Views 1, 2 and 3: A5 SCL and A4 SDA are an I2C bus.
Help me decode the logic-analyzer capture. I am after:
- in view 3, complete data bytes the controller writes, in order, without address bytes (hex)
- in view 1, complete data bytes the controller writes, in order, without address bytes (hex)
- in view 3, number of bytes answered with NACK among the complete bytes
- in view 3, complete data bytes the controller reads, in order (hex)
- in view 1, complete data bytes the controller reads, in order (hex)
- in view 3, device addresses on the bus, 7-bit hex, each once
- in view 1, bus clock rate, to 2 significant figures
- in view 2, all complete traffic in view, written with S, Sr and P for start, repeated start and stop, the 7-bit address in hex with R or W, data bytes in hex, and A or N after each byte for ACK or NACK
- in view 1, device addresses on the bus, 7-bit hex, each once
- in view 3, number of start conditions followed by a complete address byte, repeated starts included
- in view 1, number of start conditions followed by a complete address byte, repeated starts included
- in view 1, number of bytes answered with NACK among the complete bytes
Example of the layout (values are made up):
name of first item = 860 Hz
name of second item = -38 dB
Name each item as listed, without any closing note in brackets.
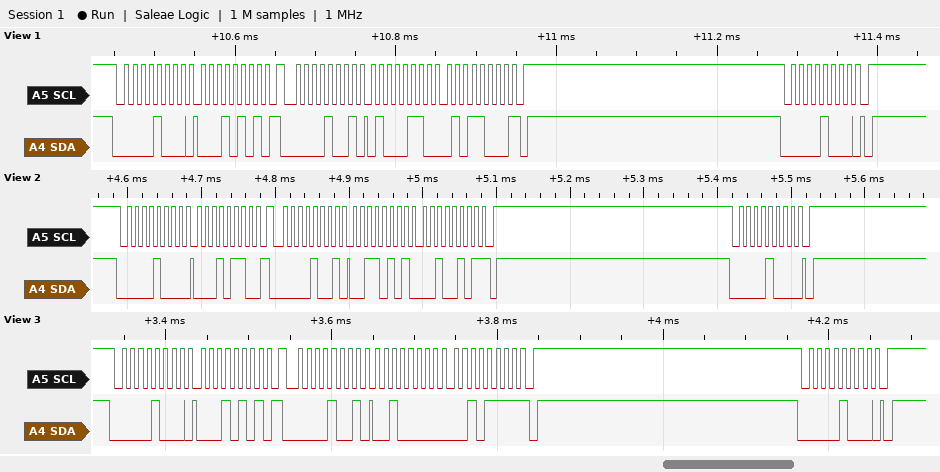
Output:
in view 3, complete data bytes the controller writes, in order, without address bytes = 15
in view 1, complete data bytes the controller writes, in order, without address bytes = 15
in view 3, number of bytes answered with NACK among the complete bytes = 1
in view 3, complete data bytes the controller reads, in order = 20 2F
in view 1, complete data bytes the controller reads, in order = 46 58
in view 3, device addresses on the bus, 7-bit hex, each once = 0x04
in view 1, bus clock rate, to 2 significant figures = 100 kHz
in view 2, all complete traffic in view, written with S, Sr and P for start, repeated start and stop, the 7-bit address in hex with R or W, data bytes in hex, and A or N after each byte for ACK or NACK = S 04W A 16 A Sr 04R A 35 A 25 N P S 04W A P
in view 1, device addresses on the bus, 7-bit hex, each once = 0x04
in view 3, number of start conditions followed by a complete address byte, repeated starts included = 3
in view 1, number of start conditions followed by a complete address byte, repeated starts included = 3
in view 1, number of bytes answered with NACK among the complete bytes = 1
